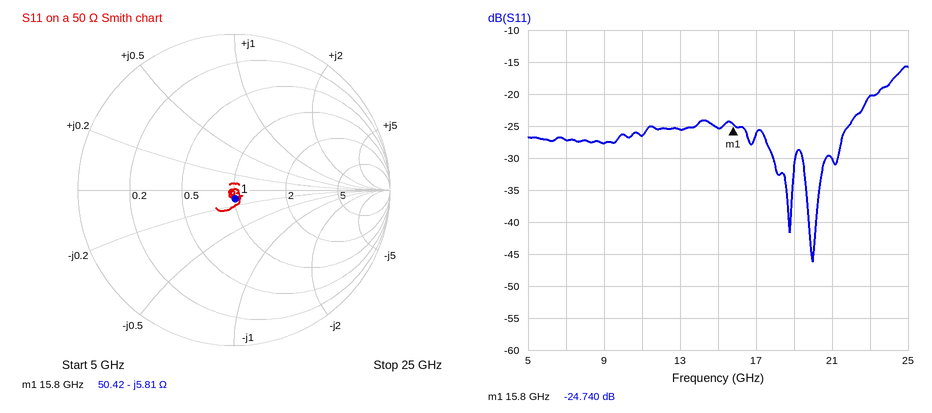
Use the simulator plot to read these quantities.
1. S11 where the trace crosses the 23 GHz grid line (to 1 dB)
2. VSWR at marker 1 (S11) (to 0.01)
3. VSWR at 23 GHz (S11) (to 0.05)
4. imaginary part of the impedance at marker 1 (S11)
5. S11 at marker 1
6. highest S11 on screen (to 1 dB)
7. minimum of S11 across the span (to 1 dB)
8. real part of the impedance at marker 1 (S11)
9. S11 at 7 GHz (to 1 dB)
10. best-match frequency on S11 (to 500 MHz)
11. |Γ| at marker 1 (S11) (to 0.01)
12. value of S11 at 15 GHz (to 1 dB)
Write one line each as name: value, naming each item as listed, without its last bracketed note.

S11 where the trace crosses the 23 GHz grid line: -20 dB
VSWR at marker 1 (S11): 1.12
VSWR at 23 GHz (S11): 1.20
imaginary part of the impedance at marker 1: -5.81 Ω
S11 at marker 1: -24.740 dB
highest S11 on screen: -16 dB
minimum of S11 across the span: -46 dB
real part of the impedance at marker 1: 50.42 Ω
S11 at 7 GHz: -27 dB
best-match frequency on S11: 20.0 GHz
|Γ| at marker 1 (S11): 0.06
value of S11 at 15 GHz: -25 dB
